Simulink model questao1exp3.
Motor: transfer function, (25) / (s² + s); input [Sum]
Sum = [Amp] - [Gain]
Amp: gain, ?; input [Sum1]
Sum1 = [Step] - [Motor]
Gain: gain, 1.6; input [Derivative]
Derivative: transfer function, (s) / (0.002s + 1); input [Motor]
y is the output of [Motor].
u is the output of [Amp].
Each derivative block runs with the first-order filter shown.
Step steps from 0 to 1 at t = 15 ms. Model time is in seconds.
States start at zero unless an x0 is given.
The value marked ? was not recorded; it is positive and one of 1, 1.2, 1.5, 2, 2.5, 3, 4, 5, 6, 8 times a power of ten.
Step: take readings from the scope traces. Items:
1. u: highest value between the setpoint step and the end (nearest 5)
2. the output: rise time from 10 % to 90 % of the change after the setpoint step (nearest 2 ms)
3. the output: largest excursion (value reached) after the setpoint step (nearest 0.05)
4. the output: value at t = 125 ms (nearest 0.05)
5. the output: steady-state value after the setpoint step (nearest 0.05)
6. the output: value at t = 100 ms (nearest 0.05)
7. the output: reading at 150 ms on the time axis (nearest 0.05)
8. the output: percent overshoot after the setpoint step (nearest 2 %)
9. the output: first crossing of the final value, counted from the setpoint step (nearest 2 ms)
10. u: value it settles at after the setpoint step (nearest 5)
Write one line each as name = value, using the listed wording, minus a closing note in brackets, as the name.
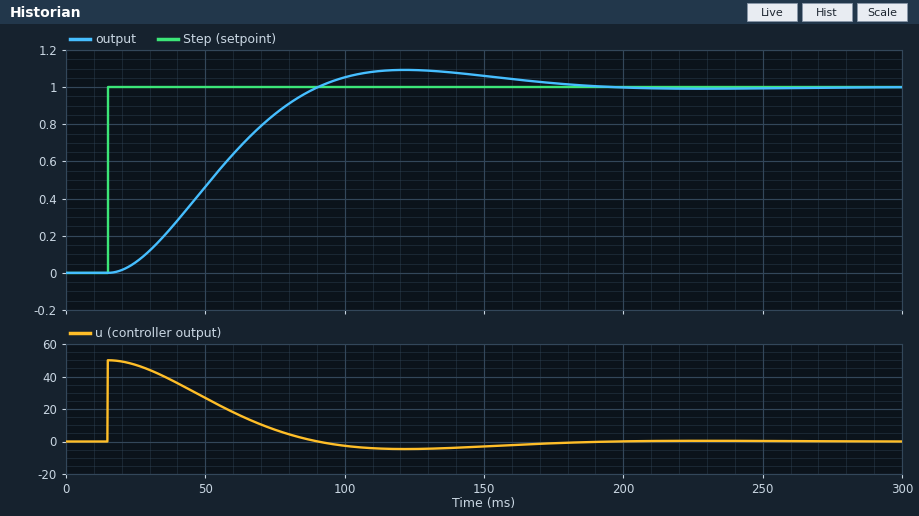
u: highest value between the setpoint step and the end = 50
the output: rise time from 10 % to 90 % of the change after the setpoint step = 50 ms
the output: largest excursion (value reached) after the setpoint step = 1.10
the output: value at t = 125 ms = 1.10
the output: steady-state value after the setpoint step = 1.00
the output: value at t = 100 ms = 1.05
the output: reading at 150 ms on the time axis = 1.05
the output: percent overshoot after the setpoint step = 10 %
the output: first crossing of the final value, counted from the setpoint step = 76 ms
u: value it settles at after the setpoint step = 0
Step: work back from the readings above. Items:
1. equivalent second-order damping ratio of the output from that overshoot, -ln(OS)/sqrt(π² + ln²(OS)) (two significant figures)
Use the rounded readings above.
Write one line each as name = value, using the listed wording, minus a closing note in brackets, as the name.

equivalent second-order damping ratio of the output from that overshoot, -ln(OS)/sqrt(π² + ln²(OS)) = 0.59
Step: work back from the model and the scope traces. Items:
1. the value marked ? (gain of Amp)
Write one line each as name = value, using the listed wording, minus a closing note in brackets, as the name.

the value marked ? = 50
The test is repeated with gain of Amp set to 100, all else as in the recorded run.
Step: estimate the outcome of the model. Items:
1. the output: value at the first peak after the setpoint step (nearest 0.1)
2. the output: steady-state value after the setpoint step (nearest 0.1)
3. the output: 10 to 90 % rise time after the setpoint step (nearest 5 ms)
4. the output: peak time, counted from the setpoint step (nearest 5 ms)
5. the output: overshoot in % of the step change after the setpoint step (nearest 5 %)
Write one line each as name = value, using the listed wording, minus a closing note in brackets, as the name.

the output: value at the first peak after the setpoint step = 1.2
the output: steady-state value after the setpoint step = 1.0
the output: 10 to 90 % rise time after the setpoint step = 30 ms
the output: peak time, counted from the setpoint step = 65 ms
the output: overshoot in % of the step change after the setpoint step = 25 %
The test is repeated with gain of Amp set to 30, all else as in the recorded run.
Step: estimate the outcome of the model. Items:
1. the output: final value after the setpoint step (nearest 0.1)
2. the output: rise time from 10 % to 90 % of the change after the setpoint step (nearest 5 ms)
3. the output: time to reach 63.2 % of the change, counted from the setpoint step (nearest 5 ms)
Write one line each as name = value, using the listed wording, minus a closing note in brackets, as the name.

the output: final value after the setpoint step = 1.0
the output: rise time from 10 % to 90 % of the change after the setpoint step = 85 ms
the output: time to reach 63.2 % of the change, counted from the setpoint step = 65 ms
